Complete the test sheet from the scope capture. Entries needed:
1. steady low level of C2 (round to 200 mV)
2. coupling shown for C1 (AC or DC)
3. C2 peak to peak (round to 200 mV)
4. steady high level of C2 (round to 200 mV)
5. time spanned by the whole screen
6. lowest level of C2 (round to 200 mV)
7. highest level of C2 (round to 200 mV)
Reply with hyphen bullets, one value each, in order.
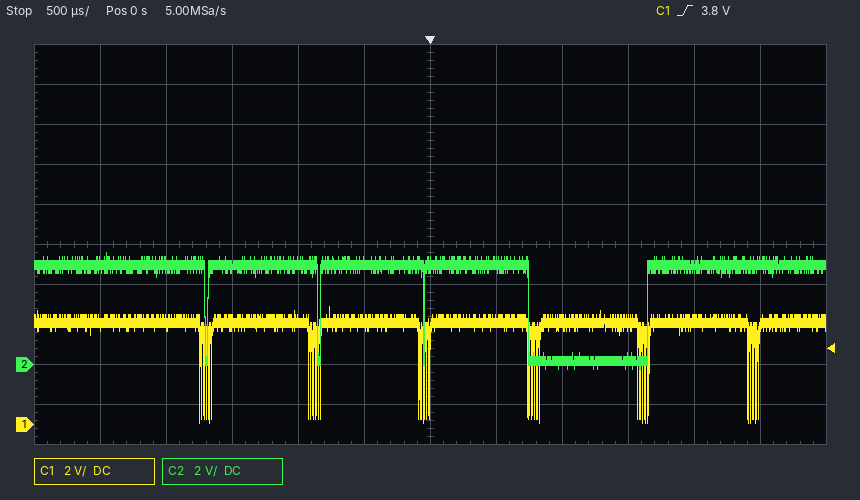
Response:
- 200 mV
- DC
- 5.8 V
- 5.0 V
- 6 ms
- -200 mV
- 5.6 V
